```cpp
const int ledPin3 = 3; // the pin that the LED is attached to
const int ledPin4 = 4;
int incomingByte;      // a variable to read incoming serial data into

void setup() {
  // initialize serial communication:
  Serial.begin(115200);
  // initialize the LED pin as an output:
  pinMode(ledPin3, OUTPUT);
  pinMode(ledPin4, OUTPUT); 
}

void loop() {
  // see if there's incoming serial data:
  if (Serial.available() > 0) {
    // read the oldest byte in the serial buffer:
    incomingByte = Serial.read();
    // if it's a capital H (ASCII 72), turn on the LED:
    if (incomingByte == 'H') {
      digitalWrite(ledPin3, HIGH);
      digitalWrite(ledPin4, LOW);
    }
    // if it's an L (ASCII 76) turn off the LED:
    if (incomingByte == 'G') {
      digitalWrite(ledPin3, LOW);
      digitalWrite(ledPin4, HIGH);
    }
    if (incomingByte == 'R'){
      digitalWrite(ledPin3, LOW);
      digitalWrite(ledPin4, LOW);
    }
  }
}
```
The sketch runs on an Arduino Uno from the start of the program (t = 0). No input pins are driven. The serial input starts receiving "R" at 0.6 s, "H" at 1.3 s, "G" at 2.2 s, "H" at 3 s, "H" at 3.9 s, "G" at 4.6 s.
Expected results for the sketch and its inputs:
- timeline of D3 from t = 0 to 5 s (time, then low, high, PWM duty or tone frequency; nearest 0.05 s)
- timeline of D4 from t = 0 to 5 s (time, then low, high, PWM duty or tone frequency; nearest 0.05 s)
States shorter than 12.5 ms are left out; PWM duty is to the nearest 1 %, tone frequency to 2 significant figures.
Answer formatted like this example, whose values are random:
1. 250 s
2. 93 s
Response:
1. 0 s low; 1.3 s high; 2.2 s low; 3 s high; 4.6 s low
2. 0 s low; 2.2 s high; 3 s low; 4.6 s high
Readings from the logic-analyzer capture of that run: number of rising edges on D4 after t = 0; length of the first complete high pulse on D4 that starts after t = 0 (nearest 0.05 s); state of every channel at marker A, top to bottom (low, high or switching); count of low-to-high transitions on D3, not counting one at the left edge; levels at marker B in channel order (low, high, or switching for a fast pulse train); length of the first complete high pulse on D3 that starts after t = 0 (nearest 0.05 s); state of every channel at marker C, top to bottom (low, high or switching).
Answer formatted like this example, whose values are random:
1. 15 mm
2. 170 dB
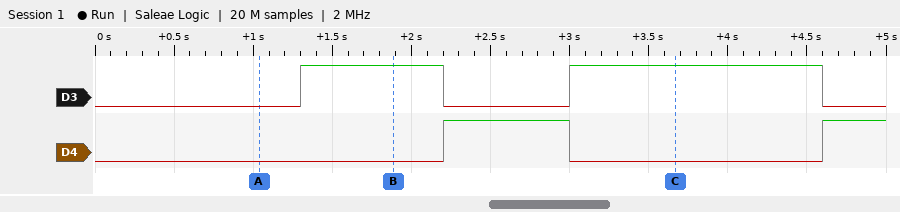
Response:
1. 2
2. 0.80 s
3. D3 low, D4 low
4. 2
5. D3 high, D4 low
6. 0.90 s
7. D3 high, D4 low
